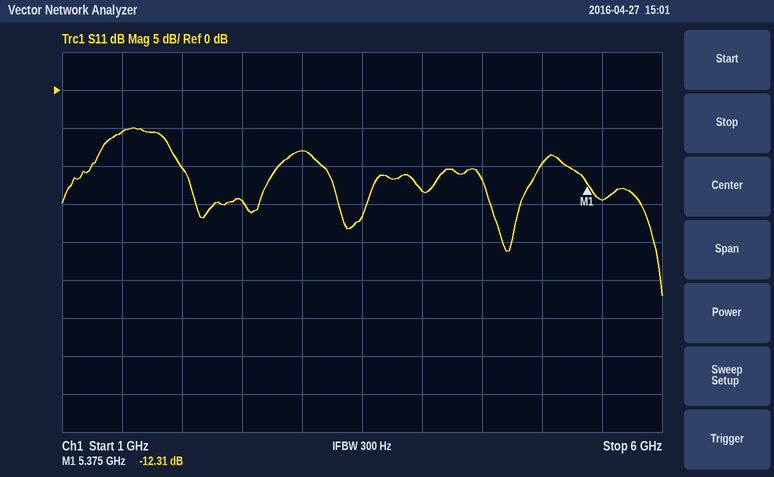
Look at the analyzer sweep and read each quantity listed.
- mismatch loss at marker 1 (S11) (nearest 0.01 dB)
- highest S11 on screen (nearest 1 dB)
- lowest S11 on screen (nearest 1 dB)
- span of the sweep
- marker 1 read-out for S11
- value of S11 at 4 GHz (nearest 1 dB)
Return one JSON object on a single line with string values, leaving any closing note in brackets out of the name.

{"mismatch loss at marker 1 (S11)": "0.26 dB", "highest S11 on screen": "-5 dB", "lowest S11 on screen": "-27 dB", "span of the sweep": "5 GHz", "marker 1 read-out for S11": "-12.31 dB", "value of S11 at 4 GHz": "-13 dB"}
